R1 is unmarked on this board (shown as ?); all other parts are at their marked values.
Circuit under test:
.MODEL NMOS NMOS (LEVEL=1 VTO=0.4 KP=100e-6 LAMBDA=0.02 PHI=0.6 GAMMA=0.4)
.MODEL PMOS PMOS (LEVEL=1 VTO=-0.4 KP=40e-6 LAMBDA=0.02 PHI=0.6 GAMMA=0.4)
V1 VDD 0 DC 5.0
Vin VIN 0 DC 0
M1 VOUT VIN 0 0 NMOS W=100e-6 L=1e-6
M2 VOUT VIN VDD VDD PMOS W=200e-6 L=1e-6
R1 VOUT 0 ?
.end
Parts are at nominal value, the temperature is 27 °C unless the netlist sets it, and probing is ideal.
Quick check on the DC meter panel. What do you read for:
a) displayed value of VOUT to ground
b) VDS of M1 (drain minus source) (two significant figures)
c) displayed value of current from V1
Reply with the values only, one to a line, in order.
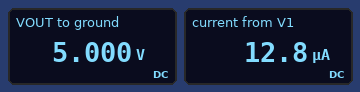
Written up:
5.000 V
5.0 V
12.8 µA
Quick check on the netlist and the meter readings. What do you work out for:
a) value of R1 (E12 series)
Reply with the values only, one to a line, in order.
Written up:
390 kΩ
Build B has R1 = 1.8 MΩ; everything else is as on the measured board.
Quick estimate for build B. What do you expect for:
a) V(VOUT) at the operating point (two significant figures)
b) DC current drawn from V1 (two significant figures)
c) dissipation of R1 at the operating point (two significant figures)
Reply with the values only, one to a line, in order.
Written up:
5.0 V
2.8 µA
14 µW
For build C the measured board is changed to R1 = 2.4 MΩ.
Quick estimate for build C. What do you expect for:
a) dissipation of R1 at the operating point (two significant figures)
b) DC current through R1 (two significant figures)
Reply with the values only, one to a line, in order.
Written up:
10 µW
2.1 µA
